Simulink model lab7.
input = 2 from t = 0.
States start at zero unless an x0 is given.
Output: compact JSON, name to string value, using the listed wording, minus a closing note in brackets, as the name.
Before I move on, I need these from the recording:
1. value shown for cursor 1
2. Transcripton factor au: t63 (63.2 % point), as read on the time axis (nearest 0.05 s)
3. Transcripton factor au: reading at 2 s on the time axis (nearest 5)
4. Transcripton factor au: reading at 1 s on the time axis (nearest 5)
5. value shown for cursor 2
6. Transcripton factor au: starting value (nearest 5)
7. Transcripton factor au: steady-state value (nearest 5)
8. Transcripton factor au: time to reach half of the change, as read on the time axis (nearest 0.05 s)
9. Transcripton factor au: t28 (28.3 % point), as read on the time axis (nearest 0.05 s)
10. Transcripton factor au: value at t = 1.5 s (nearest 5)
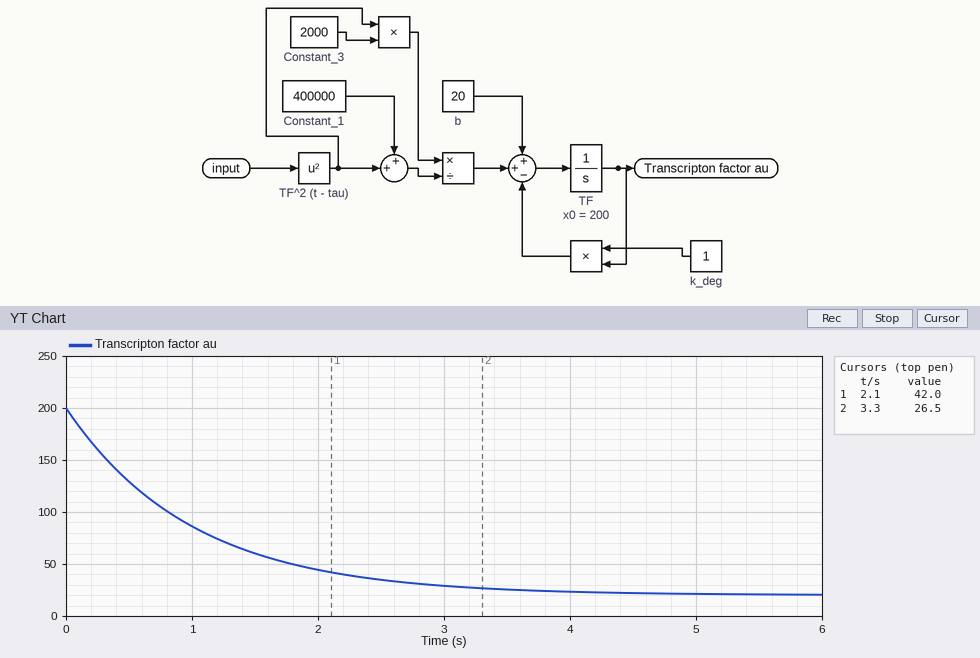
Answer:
{"value shown for cursor 1": "42.0", "Transcripton factor au: t63 (63.2 % point), as read on the time axis": "1.00 s", "Transcripton factor au: reading at 2 s on the time axis": "45", "Transcripton factor au: reading at 1 s on the time axis": "85", "value shown for cursor 2": "26.5", "Transcripton factor au: starting value": "200", "Transcripton factor au: steady-state value": "20", "Transcripton factor au: time to reach half of the change, as read on the time axis": "0.70 s", "Transcripton factor au: t28 (28.3 % point), as read on the time axis": "0.35 s", "Transcripton factor au: value at t = 1.5 s": "60"}
